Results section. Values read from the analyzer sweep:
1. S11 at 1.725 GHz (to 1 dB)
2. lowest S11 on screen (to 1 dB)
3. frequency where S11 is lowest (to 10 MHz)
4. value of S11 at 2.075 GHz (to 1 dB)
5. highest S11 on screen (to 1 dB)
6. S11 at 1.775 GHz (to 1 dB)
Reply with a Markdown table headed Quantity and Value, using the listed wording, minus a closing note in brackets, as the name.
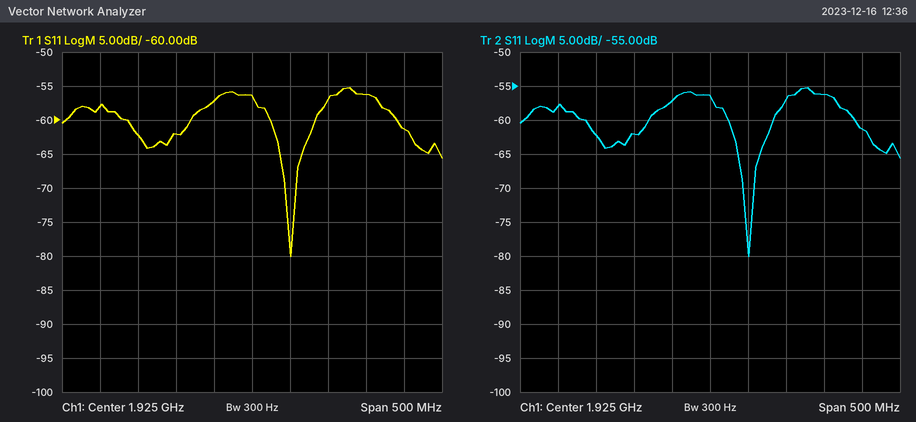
| Quantity | Value |
|---|---|
| S11 at 1.725 GHz | -58 dB |
| lowest S11 on screen | -80 dB |
| frequency where S11 is lowest | 1.98 GHz |
| value of S11 at 2.075 GHz | -56 dB |
| highest S11 on screen | -55 dB |
| S11 at 1.775 GHz | -62 dB |
